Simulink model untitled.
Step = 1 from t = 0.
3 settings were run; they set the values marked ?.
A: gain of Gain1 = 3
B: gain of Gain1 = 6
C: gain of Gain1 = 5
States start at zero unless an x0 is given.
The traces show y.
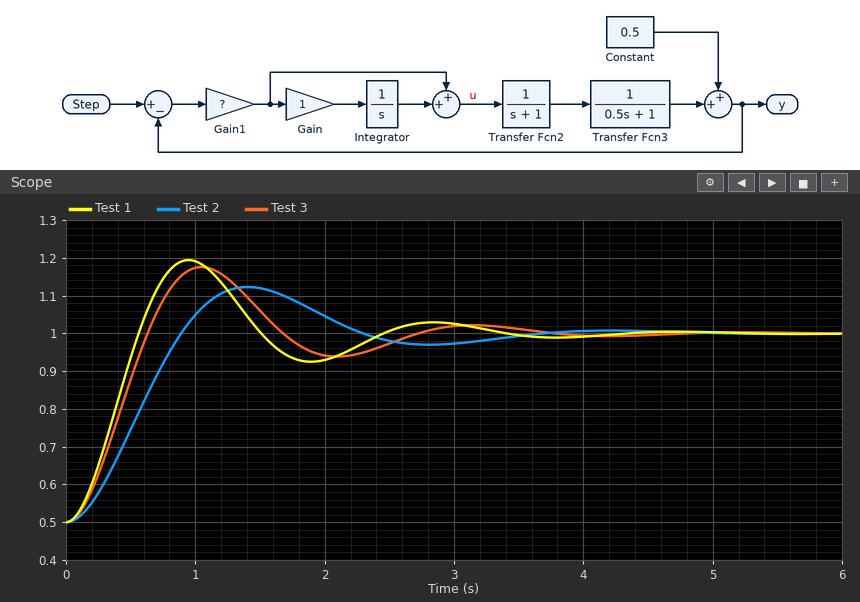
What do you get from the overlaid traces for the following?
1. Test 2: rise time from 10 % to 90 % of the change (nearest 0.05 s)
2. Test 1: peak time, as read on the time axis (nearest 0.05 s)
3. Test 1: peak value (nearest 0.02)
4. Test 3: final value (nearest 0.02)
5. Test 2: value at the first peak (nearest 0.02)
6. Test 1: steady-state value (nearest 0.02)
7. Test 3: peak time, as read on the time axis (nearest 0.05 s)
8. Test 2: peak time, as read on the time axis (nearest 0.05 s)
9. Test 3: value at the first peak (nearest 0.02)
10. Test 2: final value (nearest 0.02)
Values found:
0.60 s
0.95 s
1.20
1.00
1.12
1.00
1.05 s
1.40 s
1.18
1.00
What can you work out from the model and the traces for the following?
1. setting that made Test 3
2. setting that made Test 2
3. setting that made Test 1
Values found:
C
A
B
